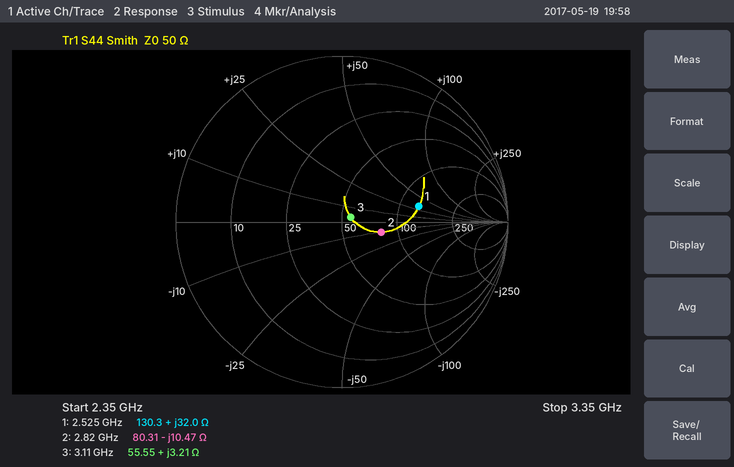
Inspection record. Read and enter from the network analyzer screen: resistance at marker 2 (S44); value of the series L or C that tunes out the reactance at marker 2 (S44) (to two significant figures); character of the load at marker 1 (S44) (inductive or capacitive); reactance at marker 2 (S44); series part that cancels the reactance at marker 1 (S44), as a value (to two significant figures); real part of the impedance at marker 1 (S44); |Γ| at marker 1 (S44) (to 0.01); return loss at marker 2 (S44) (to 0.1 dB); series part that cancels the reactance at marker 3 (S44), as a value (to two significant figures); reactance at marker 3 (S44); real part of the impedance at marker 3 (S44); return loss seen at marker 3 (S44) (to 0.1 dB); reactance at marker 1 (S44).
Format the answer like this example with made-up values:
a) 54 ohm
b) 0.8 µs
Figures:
a) 80.31 Ω
b) 590 pH
c) inductive
d) -10.47 Ω
e) 2.0 pF
f) 130.3 Ω
g) 0.47
h) 12.2 dB
i) 16 pF
j) +3.21 Ω
k) 55.55 Ω
l) 24.3 dB
m) +32.0 Ω
